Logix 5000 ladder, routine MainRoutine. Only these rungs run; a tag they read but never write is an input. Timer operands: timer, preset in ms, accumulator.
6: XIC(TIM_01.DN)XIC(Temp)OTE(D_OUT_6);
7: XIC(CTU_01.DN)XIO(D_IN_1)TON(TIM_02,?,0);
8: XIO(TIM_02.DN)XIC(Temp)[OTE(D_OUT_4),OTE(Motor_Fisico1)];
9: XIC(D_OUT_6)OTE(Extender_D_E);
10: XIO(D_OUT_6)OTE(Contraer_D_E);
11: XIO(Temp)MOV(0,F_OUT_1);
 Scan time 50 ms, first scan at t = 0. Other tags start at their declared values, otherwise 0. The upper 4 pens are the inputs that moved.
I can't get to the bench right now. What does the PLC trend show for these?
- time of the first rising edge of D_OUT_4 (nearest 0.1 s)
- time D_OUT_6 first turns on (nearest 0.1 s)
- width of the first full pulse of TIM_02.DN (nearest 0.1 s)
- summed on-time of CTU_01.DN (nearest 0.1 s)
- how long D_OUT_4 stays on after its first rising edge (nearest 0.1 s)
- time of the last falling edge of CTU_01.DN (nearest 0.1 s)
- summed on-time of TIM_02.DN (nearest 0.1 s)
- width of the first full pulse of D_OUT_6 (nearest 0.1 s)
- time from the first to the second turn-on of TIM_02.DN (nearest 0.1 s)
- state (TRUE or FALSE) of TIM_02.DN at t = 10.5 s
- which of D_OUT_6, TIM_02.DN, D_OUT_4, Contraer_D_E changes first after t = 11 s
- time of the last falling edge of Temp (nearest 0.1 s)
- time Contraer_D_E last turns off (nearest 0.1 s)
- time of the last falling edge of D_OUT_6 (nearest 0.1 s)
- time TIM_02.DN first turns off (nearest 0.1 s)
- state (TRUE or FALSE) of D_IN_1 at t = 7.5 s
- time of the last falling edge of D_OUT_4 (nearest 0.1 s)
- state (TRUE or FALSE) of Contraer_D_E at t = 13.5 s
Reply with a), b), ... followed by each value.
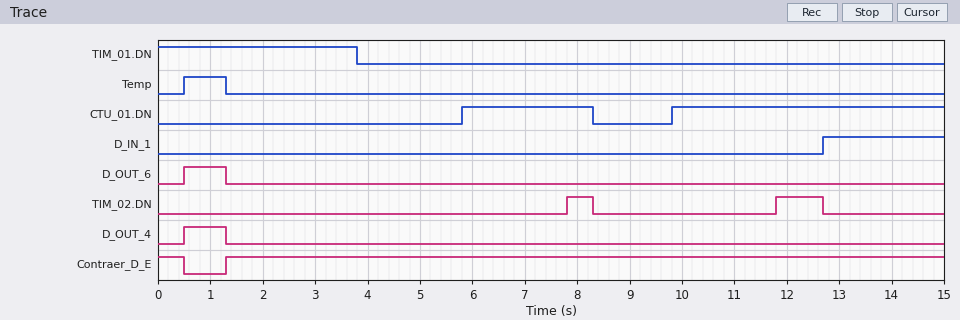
a) 0.5 s
b) 0.5 s
c) 0.5 s
d) 7.7 s
e) 0.8 s
f) 8.3 s
g) 1.4 s
h) 0.8 s
i) 4.0 s
j) FALSE
k) TIM_02.DN
l) 1.3 s
m) 0.5 s
n) 1.3 s
o) 8.3 s
p) FALSE
q) 1.3 s
r) TRUE
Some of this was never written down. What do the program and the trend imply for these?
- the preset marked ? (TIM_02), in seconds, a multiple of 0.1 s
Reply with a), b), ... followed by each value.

a) 2.0 s
